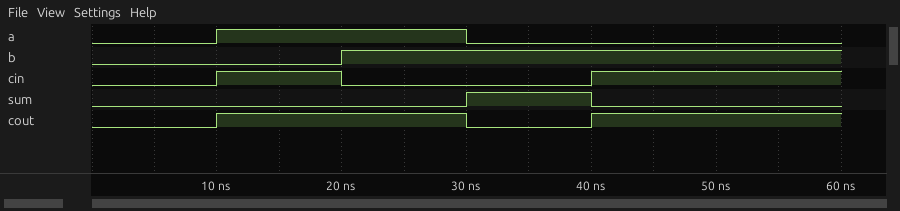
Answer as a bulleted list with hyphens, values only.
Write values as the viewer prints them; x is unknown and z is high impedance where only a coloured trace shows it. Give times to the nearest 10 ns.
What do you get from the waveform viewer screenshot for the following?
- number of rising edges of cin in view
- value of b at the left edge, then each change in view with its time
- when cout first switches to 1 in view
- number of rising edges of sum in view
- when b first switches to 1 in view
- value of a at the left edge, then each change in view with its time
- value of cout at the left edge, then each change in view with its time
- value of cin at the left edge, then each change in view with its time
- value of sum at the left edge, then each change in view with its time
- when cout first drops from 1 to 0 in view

- 2
- 0, 1 at 20 ns
- 10 ns
- 1
- 20 ns
- 0, 1 at 10 ns, 0 at 30 ns
- 0, 1 at 10 ns, 0 at 30 ns, 1 at 40 ns
- 0, 1 at 10 ns, 0 at 20 ns, 1 at 40 ns
- 0, 1 at 30 ns, 0 at 40 ns
- 30 ns
